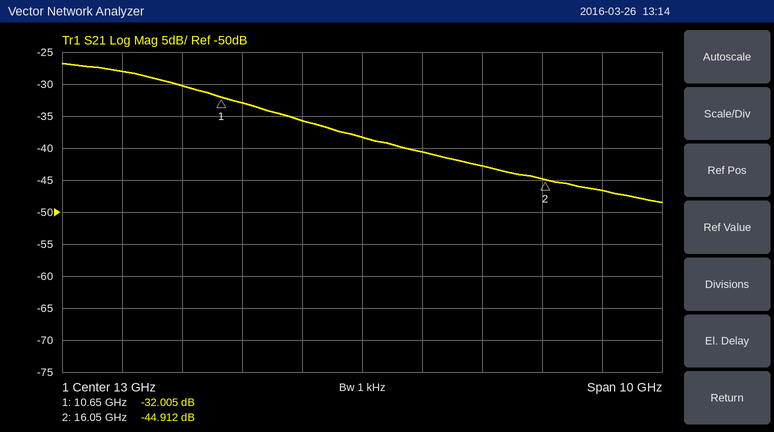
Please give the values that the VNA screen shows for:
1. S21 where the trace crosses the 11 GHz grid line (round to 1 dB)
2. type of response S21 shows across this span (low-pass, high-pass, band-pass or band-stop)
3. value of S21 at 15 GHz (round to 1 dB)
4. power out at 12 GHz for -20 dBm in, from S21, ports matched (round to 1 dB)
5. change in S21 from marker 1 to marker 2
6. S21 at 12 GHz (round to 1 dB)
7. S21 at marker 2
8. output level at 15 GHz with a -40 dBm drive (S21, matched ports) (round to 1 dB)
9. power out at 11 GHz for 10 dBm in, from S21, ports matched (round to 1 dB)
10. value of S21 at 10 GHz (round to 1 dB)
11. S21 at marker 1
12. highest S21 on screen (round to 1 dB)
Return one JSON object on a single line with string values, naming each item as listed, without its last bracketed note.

{"S21 where the trace crosses the 11 GHz grid line": "-33 dB", "type of response S21 shows across this span": "low-pass", "value of S21 at 15 GHz": "-43 dB", "power out at 12 GHz for -20 dBm in, from S21, ports matched": "-56 dBm", "change in S21 from marker 1 to marker 2": "-12.907 dB", "S21 at 12 GHz": "-36 dB", "S21 at marker 2": "-44.912 dB", "output level at 15 GHz with a -40 dBm drive (S21, matched ports)": "-83 dBm", "power out at 11 GHz for 10 dBm in, from S21, ports matched": "-23 dBm", "value of S21 at 10 GHz": "-30 dB", "S21 at marker 1": "-32.005 dB", "highest S21 on screen": "-27 dB"}
